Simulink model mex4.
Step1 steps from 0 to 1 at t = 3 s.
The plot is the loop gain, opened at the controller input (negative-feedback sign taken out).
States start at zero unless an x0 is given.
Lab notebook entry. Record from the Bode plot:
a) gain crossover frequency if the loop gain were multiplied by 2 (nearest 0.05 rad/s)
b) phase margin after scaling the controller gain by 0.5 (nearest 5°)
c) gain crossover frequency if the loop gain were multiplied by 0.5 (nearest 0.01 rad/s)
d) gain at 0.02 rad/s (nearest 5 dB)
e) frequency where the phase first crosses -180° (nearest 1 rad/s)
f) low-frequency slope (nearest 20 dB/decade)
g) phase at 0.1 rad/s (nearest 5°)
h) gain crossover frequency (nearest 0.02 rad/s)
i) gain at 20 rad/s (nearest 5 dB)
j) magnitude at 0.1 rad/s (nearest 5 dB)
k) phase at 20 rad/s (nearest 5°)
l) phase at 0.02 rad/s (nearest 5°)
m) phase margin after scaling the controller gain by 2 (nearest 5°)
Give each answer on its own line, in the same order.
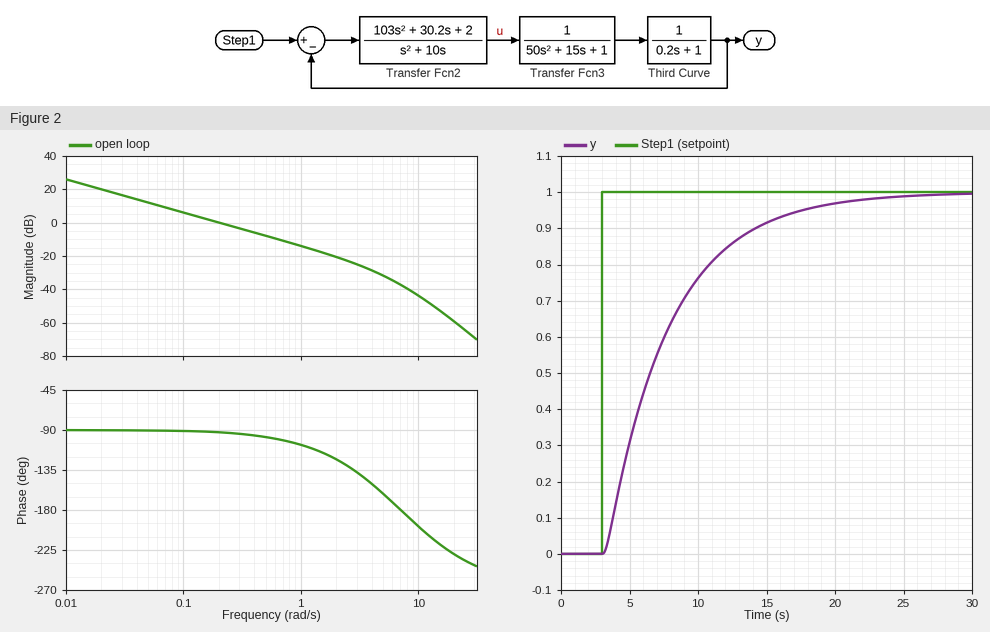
0.40 rad/s
90°
0.10 rad/s
20 dB
7 rad/s
-20 dB/decade
-90°
0.20 rad/s
-60 dB
5 dB
-230°
-90°
85°
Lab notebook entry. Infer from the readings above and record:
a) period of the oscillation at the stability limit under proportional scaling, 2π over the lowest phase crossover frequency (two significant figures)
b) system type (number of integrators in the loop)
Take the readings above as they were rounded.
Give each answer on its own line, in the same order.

0.90 s
1
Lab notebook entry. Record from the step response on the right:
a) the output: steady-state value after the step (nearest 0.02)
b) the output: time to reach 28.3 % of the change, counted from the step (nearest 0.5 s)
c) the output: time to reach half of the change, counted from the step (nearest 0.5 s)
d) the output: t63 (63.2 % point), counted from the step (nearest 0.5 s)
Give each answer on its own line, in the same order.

1.00
2.0 s
3.5 s
5.0 s
